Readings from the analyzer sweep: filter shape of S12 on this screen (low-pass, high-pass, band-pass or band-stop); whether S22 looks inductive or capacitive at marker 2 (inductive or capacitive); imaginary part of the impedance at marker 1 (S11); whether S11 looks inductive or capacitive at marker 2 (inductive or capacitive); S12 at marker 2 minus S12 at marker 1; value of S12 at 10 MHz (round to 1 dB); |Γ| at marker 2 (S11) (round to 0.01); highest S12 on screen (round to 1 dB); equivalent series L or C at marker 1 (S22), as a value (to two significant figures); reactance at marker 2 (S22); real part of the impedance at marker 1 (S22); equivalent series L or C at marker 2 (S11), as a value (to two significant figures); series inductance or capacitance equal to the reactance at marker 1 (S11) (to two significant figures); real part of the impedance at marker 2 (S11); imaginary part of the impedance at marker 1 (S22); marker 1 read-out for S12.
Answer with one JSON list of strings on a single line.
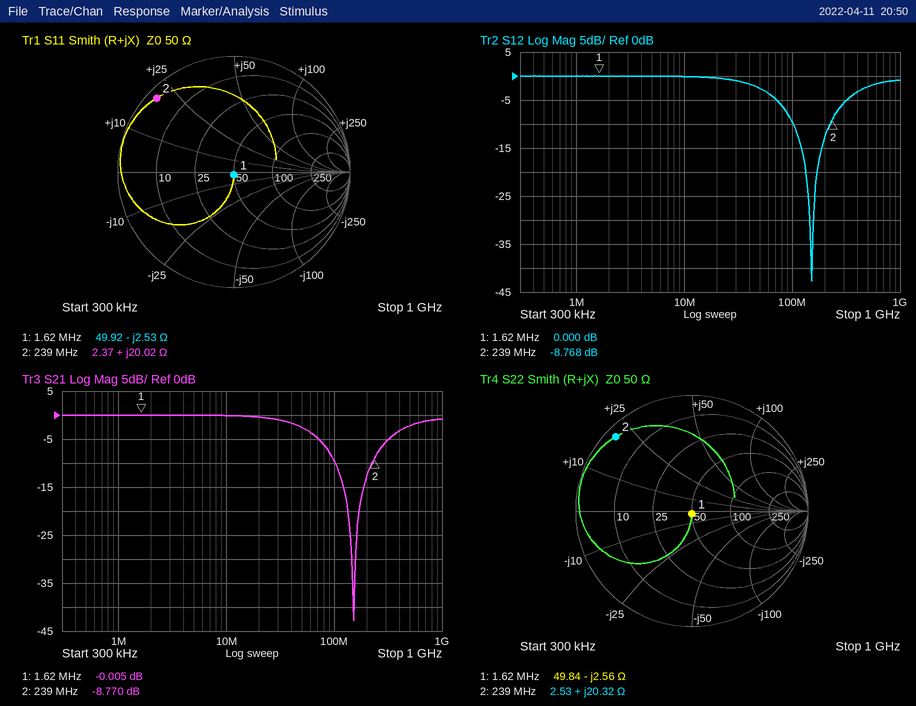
["band-stop", "inductive", "-2.53 Ω", "inductive", "-8.768 dB", "0 dB", "0.92", "0 dB", "38 nF", "+20.32 Ω", "49.84 Ω", "13 nH", "39 nF", "2.37 Ω", "-2.56 Ω", "0.000 dB"]
